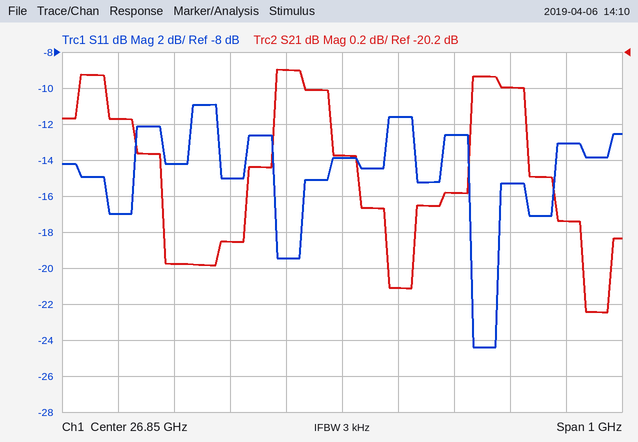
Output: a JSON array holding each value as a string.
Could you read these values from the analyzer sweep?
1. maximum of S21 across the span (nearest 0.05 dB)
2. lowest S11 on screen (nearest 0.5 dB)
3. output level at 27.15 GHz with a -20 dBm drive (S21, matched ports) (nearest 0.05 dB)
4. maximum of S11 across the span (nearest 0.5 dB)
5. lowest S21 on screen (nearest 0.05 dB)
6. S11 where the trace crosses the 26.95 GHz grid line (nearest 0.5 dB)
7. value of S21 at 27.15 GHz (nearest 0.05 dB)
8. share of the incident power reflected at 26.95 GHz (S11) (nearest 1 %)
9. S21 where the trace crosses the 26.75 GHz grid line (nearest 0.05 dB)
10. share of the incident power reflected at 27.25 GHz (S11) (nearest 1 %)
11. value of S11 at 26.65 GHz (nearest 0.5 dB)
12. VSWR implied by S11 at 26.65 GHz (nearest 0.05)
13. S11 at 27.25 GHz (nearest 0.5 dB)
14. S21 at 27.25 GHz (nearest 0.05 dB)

["-20.30 dB", "-24.5 dB", "-40.40 dBm", "-11.0 dB", "-21.65 dB", "-11.5 dB", "-20.40 dB", "7 %", "-20.30 dB", "5 %", "-15.0 dB", "1.45", "-13.0 dB", "-21.15 dB"]
